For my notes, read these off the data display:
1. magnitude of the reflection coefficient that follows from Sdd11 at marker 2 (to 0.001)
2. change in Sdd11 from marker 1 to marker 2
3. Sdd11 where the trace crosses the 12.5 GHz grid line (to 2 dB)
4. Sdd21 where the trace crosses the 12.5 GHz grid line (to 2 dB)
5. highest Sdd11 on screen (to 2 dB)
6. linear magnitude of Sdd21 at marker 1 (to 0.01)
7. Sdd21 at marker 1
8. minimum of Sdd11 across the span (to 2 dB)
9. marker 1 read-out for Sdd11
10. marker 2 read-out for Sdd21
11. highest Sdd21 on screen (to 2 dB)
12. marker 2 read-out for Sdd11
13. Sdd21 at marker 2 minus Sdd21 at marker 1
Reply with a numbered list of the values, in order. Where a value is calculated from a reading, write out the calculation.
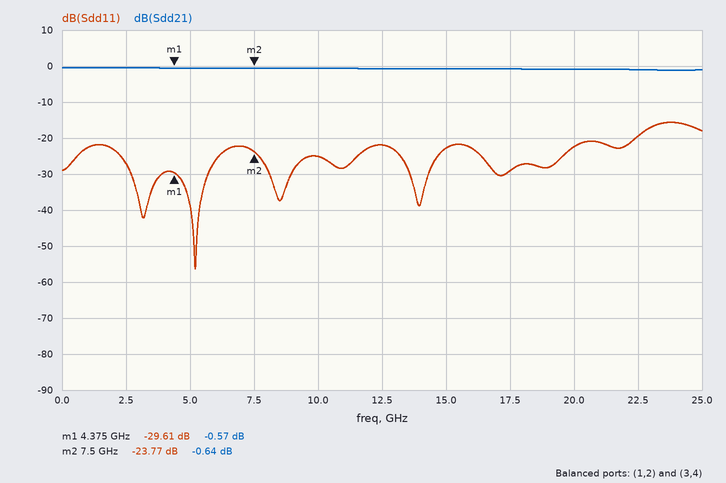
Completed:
1. 10^(-23.77/20) ≈ 0.065
2. -23.77 − (-29.61) = 5.84 dB
3. -22 dB
4. 0 dB
5. -16 dB
6. 10^(-0.57/20) ≈ 0.94
7. -0.57 dB
8. -56 dB
9. -29.61 dB
10. -0.64 dB
11. 0 dB
12. -23.77 dB
13. -0.64 − (-0.57) = -0.07 dB
